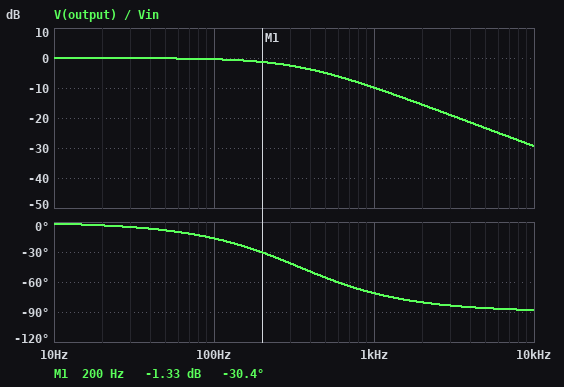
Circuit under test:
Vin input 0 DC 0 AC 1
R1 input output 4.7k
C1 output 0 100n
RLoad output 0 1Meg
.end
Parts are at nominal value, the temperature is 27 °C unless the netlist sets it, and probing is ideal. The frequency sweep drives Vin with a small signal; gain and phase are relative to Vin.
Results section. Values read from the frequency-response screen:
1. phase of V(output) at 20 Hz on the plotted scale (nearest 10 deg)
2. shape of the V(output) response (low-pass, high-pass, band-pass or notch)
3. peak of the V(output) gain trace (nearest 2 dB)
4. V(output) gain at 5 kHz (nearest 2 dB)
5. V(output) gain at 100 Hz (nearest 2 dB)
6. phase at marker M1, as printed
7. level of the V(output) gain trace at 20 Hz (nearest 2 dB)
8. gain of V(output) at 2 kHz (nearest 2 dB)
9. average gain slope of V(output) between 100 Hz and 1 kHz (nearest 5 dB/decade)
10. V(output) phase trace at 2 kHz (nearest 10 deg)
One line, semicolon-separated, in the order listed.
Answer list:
0 deg; low-pass; 0 dB; -24 dB; 0 dB; -30.4 deg; 0 dB; -16 dB; -10 dB/decade; -80 deg
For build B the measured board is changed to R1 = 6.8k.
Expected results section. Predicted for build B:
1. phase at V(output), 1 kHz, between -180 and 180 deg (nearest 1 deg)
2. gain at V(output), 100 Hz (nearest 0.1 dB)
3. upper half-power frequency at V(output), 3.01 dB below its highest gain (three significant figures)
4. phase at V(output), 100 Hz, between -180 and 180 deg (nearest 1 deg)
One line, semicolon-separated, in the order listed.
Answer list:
-77 deg; -0.8 dB; 236 Hz; -23 deg
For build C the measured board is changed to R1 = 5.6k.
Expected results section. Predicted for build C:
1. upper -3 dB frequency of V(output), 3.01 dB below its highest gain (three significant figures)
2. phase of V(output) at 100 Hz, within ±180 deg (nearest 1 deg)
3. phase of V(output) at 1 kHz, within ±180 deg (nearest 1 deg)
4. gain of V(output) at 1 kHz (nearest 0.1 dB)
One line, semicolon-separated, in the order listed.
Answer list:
286 Hz; -19 deg; -74 deg; -11.3 dB
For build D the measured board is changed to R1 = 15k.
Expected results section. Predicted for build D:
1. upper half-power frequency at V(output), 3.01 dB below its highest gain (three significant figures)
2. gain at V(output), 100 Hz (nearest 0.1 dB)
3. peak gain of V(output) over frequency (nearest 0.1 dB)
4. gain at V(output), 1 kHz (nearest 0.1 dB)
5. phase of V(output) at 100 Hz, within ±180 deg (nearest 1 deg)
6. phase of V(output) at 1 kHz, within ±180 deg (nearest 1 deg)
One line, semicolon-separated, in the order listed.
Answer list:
108 Hz; -2.8 dB; -0.1 dB; -19.5 dB; -43 deg; -84 deg
